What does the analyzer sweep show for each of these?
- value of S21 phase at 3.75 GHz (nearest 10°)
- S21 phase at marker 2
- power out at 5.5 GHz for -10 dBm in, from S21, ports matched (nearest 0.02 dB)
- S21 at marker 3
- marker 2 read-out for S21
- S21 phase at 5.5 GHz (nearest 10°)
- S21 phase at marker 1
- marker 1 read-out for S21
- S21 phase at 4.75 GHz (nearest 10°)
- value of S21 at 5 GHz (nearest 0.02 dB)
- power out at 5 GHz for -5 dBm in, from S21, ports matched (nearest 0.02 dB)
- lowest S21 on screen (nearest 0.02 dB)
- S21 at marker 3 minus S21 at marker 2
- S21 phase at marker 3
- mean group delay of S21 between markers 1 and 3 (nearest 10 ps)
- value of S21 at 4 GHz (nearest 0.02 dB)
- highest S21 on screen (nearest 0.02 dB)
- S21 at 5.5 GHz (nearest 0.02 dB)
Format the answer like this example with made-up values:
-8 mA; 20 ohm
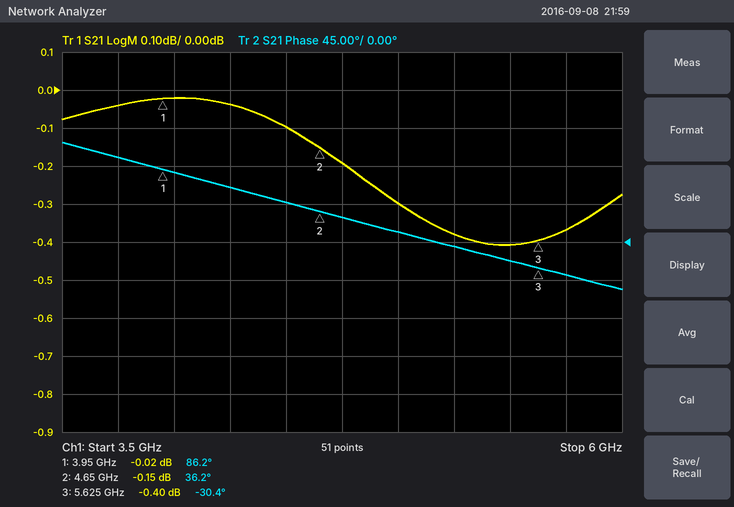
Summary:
100°; 36.2°; -10.40 dBm; -0.40 dB; -0.15 dB; -20°; 86.2°; -0.02 dB; 30°; -0.30 dB; -5.30 dBm; -0.40 dB; -0.25 dB; -30.4°; 190 ps; -0.02 dB; -0.02 dB; -0.40 dB
